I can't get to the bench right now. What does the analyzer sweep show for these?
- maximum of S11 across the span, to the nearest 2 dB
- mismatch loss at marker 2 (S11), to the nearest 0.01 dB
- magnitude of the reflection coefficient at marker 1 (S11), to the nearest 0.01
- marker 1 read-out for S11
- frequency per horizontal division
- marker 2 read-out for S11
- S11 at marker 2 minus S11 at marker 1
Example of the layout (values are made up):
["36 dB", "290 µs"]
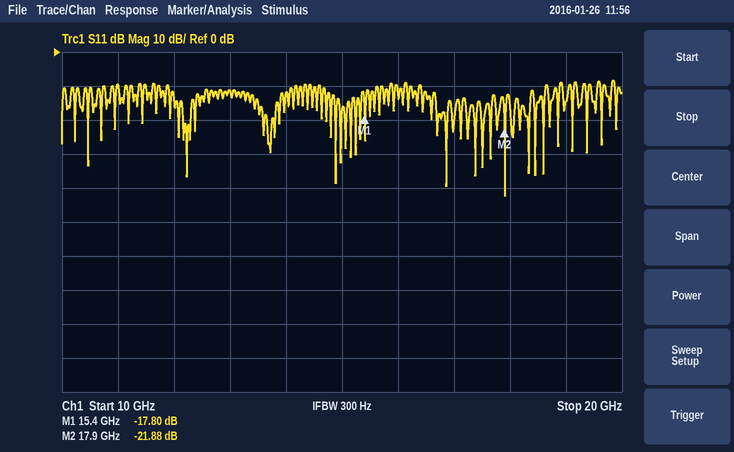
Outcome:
["-8 dB", "0.03 dB", "0.13", "-17.80 dB", "1 GHz", "-21.88 dB", "-4.08 dB"]
